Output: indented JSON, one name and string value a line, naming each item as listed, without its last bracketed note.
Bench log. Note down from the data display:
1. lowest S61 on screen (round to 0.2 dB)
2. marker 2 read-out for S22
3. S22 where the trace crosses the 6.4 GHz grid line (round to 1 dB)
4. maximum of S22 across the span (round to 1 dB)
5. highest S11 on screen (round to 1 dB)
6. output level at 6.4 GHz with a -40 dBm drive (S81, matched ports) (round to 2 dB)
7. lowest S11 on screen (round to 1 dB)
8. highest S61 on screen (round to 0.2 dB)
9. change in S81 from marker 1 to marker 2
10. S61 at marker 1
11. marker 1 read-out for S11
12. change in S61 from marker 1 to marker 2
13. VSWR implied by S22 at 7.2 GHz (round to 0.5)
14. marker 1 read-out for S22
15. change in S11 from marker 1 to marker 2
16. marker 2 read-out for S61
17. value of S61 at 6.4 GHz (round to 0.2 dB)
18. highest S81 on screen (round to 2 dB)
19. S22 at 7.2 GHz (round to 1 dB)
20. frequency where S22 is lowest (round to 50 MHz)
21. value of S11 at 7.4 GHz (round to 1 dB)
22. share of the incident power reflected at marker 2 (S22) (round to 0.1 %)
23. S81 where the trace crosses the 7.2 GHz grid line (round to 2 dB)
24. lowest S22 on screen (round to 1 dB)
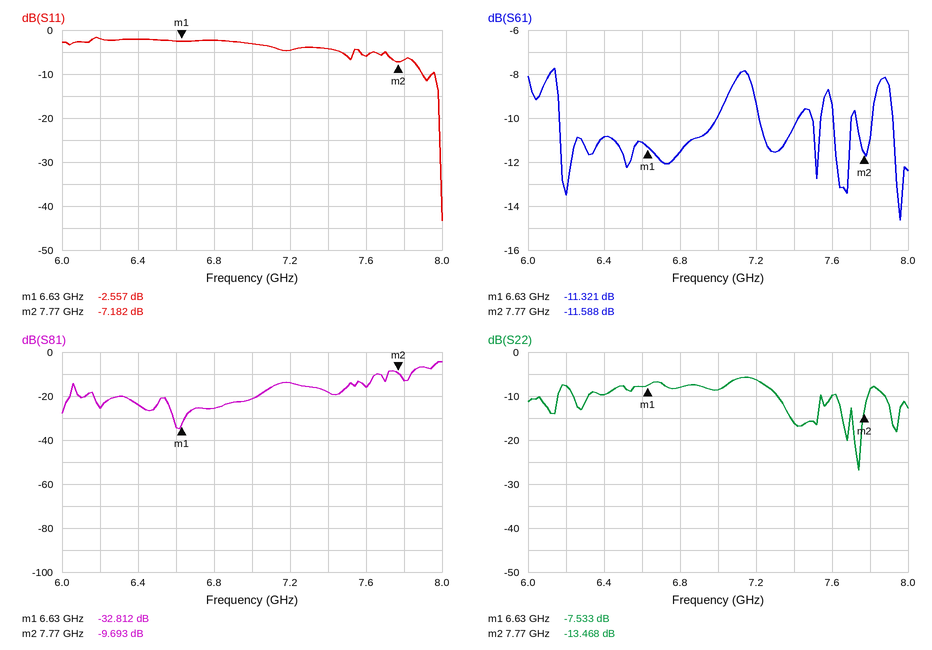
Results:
{
  "lowest S61 on screen": "-14.6 dB",
  "marker 2 read-out for S22": "-13.468 dB",
  "S22 where the trace crosses the 6.4 GHz grid line": "-10 dB",
  "maximum of S22 across the span": "-6 dB",
  "highest S11 on screen": "-2 dB",
  "output level at 6.4 GHz with a -40 dBm drive (S81, matched ports)": "-64 dBm",
  "lowest S11 on screen": "-43 dB",
  "highest S61 on screen": "-7.8 dB",
  "change in S81 from marker 1 to marker 2": "23.119 dB",
  "S61 at marker 1": "-11.321 dB",
  "marker 1 read-out for S11": "-2.557 dB",
  "change in S61 from marker 1 to marker 2": "-0.267 dB",
  "VSWR implied by S22 at 7.2 GHz": "3.0",
  "marker 1 read-out for S22": "-7.533 dB",
  "change in S11 from marker 1 to marker 2": "-4.625 dB",
  "marker 2 read-out for S61": "-11.588 dB",
  "value of S61 at 6.4 GHz": "-10.8 dB",
  "highest S81 on screen": "-4 dB",
  "S22 at 7.2 GHz": "-6 dB",
  "frequency where S22 is lowest": "7.75 GHz",
  "value of S11 at 7.4 GHz": "-4 dB",
  "share of the incident power reflected at marker 2 (S22)": "4.5 %",
  "S81 where the trace crosses the 7.2 GHz grid line": "-14 dB",
  "lowest S22 on screen": "-27 dB"
}
